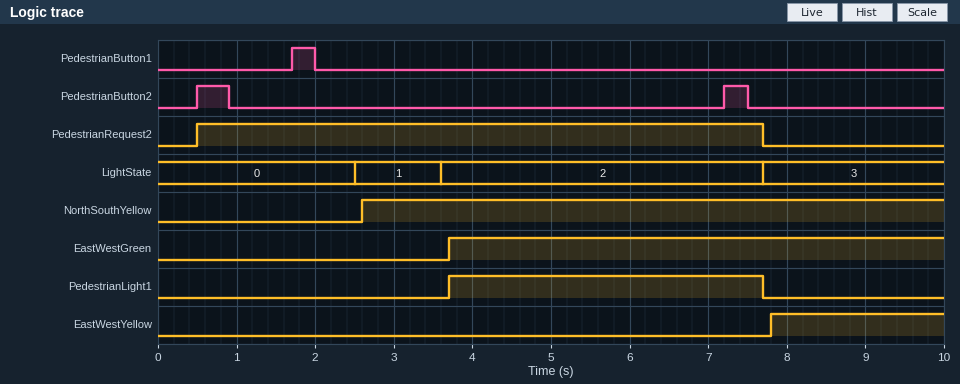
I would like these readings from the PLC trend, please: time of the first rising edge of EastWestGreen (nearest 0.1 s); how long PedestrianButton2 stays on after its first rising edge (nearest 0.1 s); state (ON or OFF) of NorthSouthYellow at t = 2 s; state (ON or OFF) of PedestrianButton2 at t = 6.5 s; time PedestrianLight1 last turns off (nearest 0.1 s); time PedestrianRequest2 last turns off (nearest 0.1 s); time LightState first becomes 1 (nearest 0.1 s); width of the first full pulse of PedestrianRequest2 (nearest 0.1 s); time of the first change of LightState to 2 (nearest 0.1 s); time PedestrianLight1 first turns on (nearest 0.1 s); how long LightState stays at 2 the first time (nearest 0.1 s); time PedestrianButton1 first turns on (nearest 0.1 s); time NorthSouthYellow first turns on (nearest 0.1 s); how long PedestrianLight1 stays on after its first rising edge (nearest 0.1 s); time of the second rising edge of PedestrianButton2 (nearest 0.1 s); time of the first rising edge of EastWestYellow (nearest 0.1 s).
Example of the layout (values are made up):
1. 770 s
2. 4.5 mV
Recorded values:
1. 3.7 s
2. 0.4 s
3. OFF
4. OFF
5. 7.7 s
6. 7.7 s
7. 2.5 s
8. 7.2 s
9. 3.6 s
10. 3.7 s
11. 4.1 s
12. 1.7 s
13. 2.6 s
14. 4.0 s
15. 7.2 s
16. 7.8 s
